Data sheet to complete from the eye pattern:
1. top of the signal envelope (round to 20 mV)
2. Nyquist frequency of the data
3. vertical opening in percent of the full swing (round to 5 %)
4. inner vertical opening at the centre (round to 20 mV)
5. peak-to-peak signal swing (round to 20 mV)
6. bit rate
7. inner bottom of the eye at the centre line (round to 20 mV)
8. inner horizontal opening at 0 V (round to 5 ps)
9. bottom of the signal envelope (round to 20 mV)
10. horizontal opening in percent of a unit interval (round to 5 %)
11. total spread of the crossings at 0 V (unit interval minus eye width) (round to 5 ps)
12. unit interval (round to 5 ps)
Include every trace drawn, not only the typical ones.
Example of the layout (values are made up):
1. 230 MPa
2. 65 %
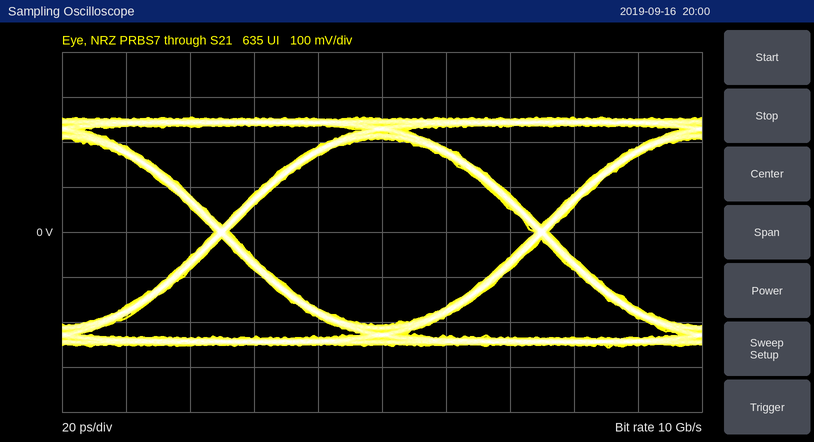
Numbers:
1. 260 mV
2. 5 GHz
3. 80 %
4. 420 mV
5. 520 mV
6. 10 Gb/s
7. -200 mV
8. 95 ps
9. -260 mV
10. 95 %
11. 5 ps
12. 100 ps
